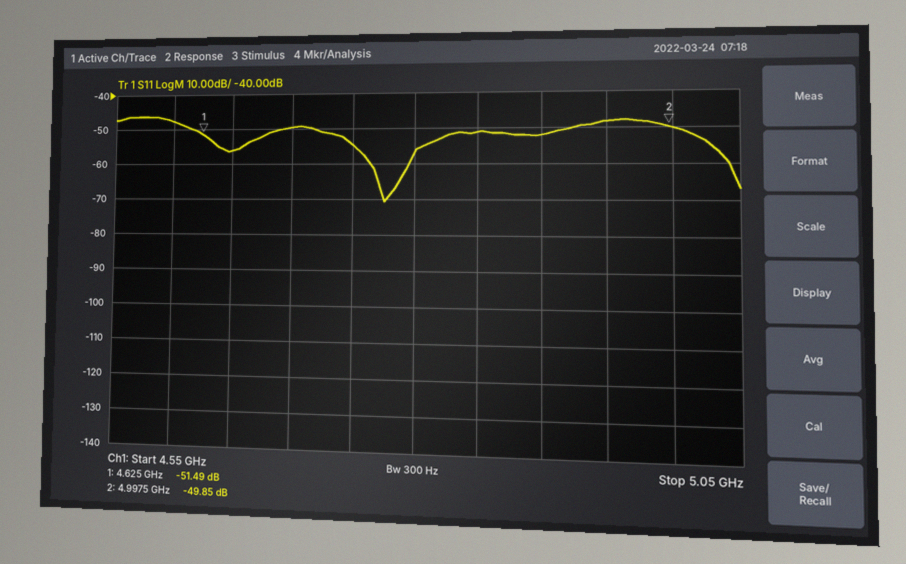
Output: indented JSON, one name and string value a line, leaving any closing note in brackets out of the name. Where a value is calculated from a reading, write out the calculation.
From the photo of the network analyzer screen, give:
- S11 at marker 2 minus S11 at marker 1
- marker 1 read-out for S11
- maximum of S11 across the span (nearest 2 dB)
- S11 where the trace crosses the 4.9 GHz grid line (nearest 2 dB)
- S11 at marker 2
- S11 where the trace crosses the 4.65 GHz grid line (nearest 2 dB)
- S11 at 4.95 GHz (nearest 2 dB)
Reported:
{
  "S11 at marker 2 minus S11 at marker 1": "-49.85 − (-51.49) = 1.64 dB",
  "marker 1 read-out for S11": "-51.49 dB",
  "maximum of S11 across the span": "-46 dB",
  "S11 where the trace crosses the 4.9 GHz grid line": "-52 dB",
  "S11 at marker 2": "-49.85 dB",
  "S11 where the trace crosses the 4.65 GHz grid line": "-56 dB",
  "S11 at 4.95 GHz": "-48 dB"
}
